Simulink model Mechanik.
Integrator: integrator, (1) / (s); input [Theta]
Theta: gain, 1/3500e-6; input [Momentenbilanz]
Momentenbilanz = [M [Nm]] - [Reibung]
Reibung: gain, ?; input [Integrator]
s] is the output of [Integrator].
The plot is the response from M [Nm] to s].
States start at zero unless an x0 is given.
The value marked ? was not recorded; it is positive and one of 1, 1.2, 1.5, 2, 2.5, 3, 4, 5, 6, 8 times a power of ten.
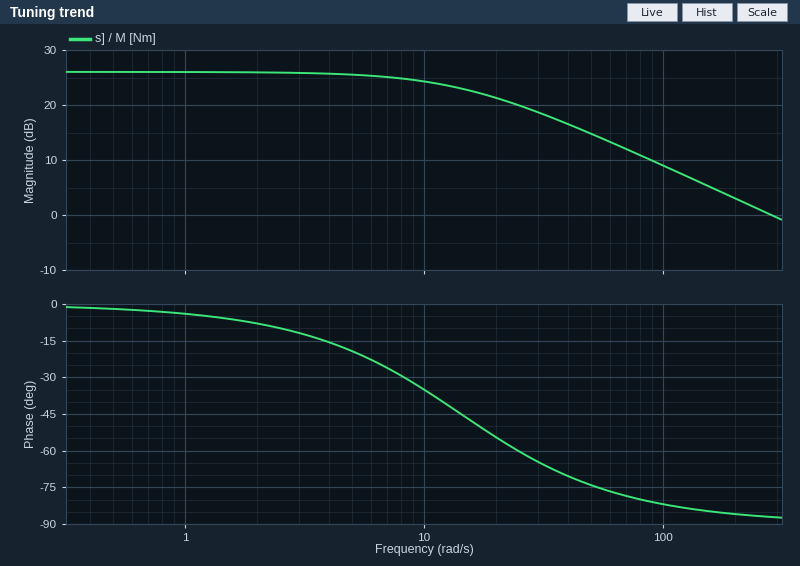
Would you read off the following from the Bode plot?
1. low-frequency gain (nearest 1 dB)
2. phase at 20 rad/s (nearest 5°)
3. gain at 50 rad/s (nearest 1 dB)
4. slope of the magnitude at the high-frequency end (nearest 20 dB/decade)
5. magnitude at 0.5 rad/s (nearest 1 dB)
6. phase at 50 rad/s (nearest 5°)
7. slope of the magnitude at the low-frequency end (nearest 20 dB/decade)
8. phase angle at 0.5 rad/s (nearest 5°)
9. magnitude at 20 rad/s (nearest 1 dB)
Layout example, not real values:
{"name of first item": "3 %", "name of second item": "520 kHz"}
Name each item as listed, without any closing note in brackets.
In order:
{"low-frequency gain": "26 dB", "phase at 20 rad/s": "-55°", "gain at 50 rad/s": "15 dB", "slope of the magnitude at the high-frequency end": "-20 dB/decade", "magnitude at 0.5 rad/s": "26 dB", "phase at 50 rad/s": "-75°", "slope of the magnitude at the low-frequency end": "0 dB/decade", "phase angle at 0.5 rad/s": "0°", "magnitude at 20 rad/s": "21 dB"}
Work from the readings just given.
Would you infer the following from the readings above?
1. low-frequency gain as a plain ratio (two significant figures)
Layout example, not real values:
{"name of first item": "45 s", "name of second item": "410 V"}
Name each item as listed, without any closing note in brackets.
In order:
{"low-frequency gain as a plain ratio": "20"}
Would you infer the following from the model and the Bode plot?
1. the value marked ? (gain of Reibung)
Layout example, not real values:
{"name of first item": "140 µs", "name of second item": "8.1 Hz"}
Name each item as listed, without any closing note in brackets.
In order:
{"the value marked ?": "0.05"}
